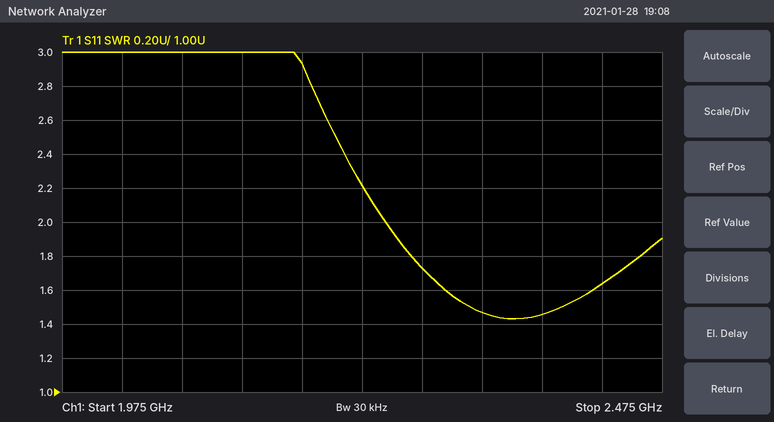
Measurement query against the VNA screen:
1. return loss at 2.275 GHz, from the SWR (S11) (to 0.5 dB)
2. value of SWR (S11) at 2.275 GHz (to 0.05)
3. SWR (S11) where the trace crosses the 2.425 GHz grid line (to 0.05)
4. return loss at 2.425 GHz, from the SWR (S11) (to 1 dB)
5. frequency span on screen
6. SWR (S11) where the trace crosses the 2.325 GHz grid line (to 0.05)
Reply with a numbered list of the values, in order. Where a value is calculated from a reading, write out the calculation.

1. −20 log10((1.75 − 1)/(1.75 + 1)) ≈ 11.3 dB, so 11.5 dB to the nearest 0.5 dB
2. 1.75
3. 1.65
4. −20 log10((1.65 − 1)/(1.65 + 1)) ≈ 12 dB
5. 500 MHz
6. 1.45
